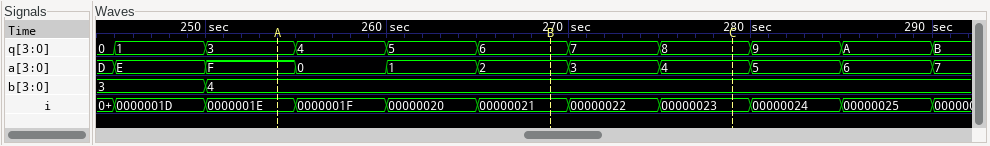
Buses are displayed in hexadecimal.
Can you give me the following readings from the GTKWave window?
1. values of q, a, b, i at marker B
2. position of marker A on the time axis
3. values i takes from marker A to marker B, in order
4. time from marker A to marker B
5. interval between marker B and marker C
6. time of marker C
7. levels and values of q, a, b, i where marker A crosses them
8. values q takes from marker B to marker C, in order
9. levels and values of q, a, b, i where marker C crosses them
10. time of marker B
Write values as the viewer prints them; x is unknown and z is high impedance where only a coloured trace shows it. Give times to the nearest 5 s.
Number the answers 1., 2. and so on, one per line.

1. q=6, a=2, b=4, i=00000021
2. 255 s
3. 0000001E, 0000001F, 00000020, 00000021
4. 15 s
5. 10 s
6. 280 s
7. q=3, a=F, b=4, i=0000001E
8. 6, 7, 8
9. q=8, a=4, b=4, i=00000023
10. 270 s
